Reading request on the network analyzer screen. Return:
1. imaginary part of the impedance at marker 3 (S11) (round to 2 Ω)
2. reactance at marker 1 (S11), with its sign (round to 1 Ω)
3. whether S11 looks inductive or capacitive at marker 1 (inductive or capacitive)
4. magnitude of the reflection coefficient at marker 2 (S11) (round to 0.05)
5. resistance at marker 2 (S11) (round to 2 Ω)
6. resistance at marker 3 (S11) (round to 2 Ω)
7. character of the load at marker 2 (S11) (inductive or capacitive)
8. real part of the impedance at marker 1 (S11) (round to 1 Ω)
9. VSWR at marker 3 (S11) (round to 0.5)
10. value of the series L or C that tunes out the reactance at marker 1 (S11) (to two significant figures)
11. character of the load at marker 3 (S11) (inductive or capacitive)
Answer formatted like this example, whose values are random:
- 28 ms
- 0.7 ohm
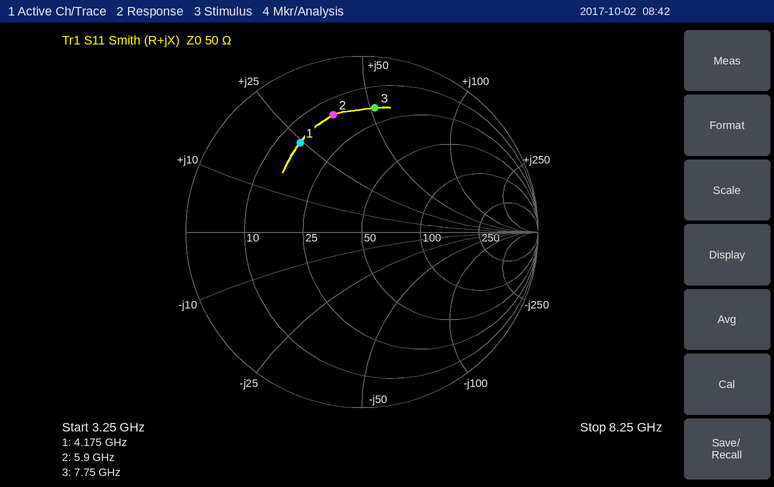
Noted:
- +52 Ω
- +24 Ω
- inductive
- 0.70
- 14 Ω
- 18 Ω
- inductive
- 15 Ω
- 6.0
- 1.6 pF
- inductive
